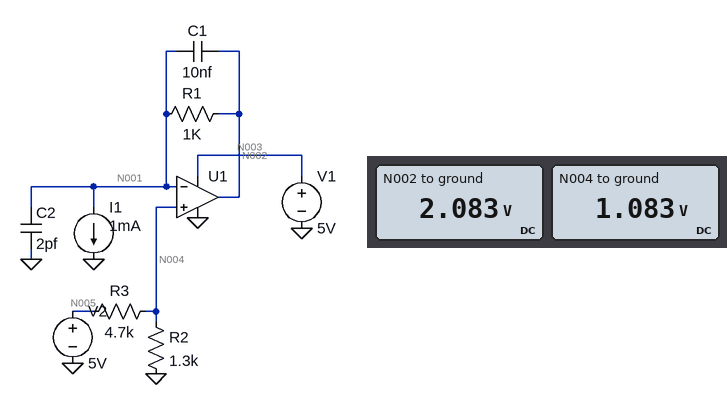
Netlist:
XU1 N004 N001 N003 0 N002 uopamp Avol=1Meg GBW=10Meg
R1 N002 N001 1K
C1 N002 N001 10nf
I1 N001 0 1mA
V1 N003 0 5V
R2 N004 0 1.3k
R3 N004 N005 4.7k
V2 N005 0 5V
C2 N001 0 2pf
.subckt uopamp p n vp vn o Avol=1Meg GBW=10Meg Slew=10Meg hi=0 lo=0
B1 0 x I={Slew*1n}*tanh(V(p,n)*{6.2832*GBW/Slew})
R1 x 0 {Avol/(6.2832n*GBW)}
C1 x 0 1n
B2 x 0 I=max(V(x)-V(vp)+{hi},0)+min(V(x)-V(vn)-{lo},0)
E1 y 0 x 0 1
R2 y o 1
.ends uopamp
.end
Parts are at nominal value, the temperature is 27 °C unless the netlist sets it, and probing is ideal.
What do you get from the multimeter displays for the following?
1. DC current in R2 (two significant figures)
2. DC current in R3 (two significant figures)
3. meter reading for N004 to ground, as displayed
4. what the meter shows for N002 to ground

830 µA
830 µA
1.083 V
2.083 V
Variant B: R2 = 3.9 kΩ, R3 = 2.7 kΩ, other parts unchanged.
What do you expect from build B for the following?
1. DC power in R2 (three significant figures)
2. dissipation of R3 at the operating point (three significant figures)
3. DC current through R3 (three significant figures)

2.24 mW
1.55 mW
758 µA
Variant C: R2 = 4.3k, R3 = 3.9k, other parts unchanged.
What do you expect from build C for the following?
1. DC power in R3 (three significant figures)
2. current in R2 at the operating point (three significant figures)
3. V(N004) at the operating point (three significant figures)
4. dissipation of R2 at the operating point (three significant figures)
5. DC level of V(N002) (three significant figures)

1.45 mW
610 µA
2.62 V
1.60 mW
3.62 V
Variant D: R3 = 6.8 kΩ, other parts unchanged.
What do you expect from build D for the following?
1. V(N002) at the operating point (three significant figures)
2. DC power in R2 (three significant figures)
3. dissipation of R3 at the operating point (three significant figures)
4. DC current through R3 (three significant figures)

1.80 V
495 µW
2.59 mW
617 µA
